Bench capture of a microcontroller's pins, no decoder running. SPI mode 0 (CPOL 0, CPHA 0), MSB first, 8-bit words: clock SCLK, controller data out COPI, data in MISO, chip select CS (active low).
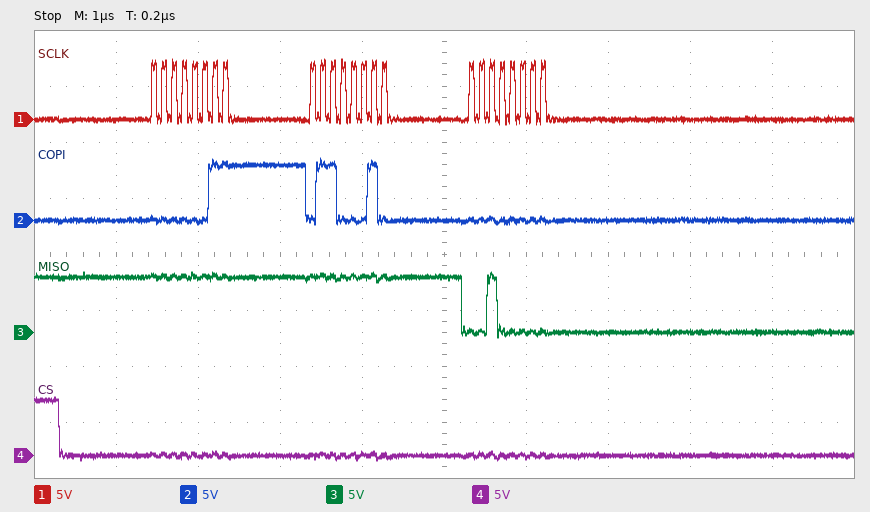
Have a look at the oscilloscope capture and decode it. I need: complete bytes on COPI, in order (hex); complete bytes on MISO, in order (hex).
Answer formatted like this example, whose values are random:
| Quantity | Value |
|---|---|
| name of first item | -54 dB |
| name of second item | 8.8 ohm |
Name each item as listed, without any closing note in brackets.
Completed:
| Quantity | Value |
|---|---|
| complete bytes on COPI, in order | 0x03 0x62 0x00 |
| complete bytes on MISO, in order | 0xFF 0xFF 0x20 |
